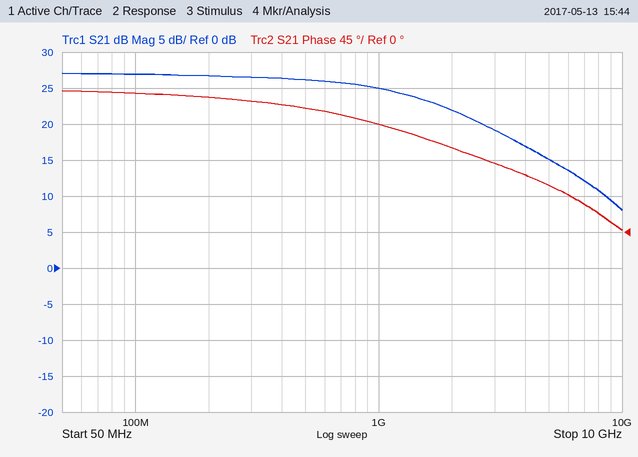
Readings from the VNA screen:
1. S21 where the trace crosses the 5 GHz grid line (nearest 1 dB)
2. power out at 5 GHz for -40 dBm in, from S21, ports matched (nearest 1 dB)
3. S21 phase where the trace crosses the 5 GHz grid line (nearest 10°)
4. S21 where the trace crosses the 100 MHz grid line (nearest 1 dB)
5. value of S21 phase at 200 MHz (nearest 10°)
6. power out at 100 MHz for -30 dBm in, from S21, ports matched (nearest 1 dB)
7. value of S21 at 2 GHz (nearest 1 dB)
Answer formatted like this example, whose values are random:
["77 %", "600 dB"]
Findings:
["15 dB", "-25 dBm", "60°", "27 dB", "170°", "-3 dBm", "22 dB"]
